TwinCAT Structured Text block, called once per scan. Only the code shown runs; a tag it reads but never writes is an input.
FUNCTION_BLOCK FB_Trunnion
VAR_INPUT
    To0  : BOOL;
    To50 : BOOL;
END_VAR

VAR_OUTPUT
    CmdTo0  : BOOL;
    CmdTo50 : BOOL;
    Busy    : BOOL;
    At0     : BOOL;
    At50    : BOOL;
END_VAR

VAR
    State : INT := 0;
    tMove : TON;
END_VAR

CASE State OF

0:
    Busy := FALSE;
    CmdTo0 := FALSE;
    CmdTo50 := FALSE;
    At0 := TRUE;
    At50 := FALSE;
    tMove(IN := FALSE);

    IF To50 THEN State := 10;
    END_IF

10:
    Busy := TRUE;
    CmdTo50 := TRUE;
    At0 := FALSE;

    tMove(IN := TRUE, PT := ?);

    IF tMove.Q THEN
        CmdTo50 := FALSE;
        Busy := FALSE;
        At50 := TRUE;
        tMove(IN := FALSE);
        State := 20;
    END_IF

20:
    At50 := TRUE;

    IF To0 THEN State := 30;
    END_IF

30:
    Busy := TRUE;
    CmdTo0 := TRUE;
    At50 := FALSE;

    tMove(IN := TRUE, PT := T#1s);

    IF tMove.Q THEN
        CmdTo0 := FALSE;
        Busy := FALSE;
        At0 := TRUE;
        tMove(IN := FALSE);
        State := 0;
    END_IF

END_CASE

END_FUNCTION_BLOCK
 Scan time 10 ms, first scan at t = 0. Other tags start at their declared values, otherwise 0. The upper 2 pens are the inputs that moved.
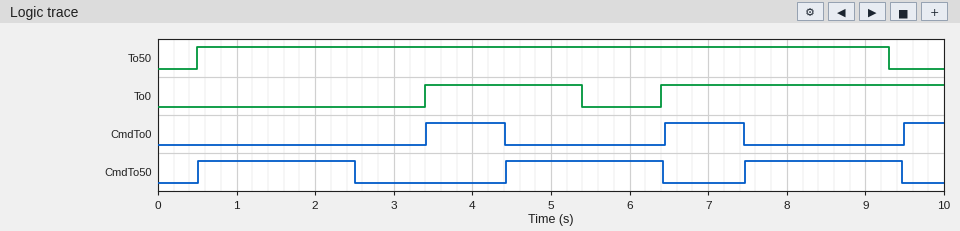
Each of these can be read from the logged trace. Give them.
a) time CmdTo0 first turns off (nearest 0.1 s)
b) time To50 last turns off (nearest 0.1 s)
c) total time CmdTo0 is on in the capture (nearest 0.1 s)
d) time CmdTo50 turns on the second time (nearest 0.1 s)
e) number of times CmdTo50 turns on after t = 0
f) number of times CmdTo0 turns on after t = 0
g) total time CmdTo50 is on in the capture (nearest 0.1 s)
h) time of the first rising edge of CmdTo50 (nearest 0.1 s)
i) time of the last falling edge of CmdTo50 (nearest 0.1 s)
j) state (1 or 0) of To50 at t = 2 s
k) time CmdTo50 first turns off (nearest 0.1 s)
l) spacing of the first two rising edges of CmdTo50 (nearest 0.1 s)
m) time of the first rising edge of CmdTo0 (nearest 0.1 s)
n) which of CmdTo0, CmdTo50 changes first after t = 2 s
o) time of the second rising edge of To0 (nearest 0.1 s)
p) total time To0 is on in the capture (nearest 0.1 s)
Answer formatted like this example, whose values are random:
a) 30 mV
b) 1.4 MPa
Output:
a) 4.4 s
b) 9.3 s
c) 2.5 s
d) 4.4 s
e) 3
f) 3
g) 6.0 s
h) 0.5 s
i) 9.5 s
j) 1
k) 2.5 s
l) 3.9 s
m) 3.4 s
n) CmdTo50
o) 6.4 s
p) 5.6 s
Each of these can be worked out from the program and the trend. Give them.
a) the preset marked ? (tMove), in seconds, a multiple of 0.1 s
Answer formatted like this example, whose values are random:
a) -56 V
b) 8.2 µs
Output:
a) 2.0 s
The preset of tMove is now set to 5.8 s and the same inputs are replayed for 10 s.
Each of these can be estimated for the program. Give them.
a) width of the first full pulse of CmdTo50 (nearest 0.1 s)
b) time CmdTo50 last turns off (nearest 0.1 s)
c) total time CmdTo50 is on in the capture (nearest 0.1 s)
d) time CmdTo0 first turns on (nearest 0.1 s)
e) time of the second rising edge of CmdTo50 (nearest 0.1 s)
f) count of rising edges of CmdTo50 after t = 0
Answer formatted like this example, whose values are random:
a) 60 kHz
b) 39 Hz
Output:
a) 5.8 s
b) 6.3 s
c) 8.4 s
d) 6.4 s
e) 7.4 s
f) 2
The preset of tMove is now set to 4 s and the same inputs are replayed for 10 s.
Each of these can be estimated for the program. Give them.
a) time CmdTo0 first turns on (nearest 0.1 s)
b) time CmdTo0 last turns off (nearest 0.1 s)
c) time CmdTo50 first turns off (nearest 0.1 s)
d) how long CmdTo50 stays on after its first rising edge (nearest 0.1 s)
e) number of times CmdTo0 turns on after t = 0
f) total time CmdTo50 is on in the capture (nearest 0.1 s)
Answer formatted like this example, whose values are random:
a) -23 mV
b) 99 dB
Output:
a) 4.5 s
b) 5.5 s
c) 4.5 s
d) 4.0 s
e) 2
f) 8.0 s
